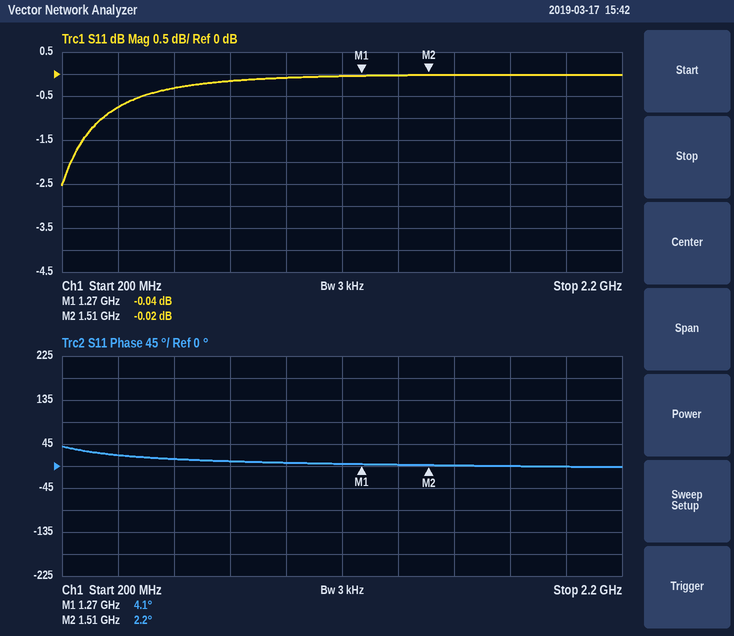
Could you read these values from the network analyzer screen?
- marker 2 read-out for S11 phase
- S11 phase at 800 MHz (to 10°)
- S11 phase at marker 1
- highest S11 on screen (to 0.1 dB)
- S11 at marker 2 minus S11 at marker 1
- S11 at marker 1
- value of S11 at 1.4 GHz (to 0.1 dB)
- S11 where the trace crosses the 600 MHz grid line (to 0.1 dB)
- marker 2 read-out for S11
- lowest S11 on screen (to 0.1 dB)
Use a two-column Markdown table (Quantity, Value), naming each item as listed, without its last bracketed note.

| Quantity | Value |
|---|---|
| marker 2 read-out for S11 phase | 2.2° |
| S11 phase at 800 MHz | 10° |
| S11 phase at marker 1 | 4.1° |
| highest S11 on screen | 0.0 dB |
| S11 at marker 2 minus S11 at marker 1 | 0.02 dB |
| S11 at marker 1 | -0.04 dB |
| value of S11 at 1.4 GHz | 0.0 dB |
| S11 where the trace crosses the 600 MHz grid line | -0.3 dB |
| marker 2 read-out for S11 | -0.02 dB |
| lowest S11 on screen | -2.5 dB |
